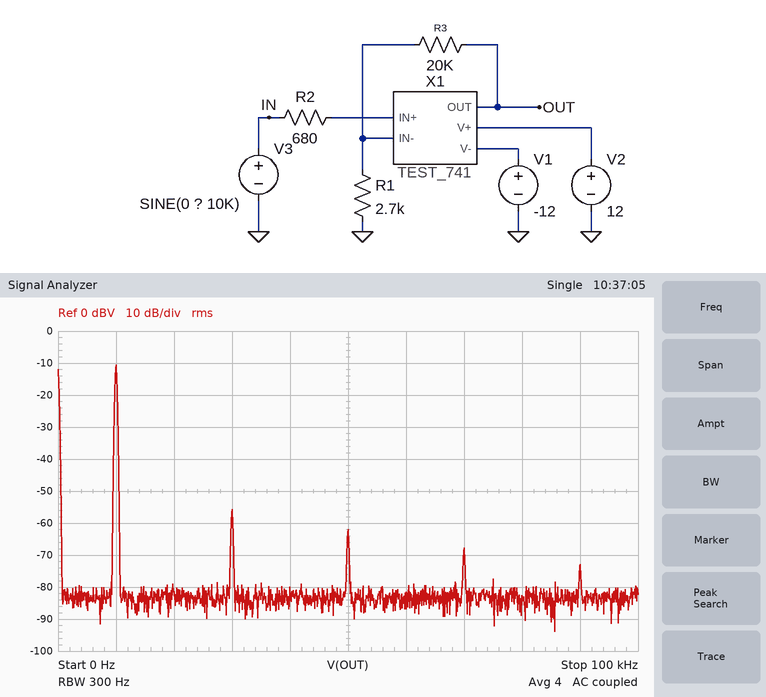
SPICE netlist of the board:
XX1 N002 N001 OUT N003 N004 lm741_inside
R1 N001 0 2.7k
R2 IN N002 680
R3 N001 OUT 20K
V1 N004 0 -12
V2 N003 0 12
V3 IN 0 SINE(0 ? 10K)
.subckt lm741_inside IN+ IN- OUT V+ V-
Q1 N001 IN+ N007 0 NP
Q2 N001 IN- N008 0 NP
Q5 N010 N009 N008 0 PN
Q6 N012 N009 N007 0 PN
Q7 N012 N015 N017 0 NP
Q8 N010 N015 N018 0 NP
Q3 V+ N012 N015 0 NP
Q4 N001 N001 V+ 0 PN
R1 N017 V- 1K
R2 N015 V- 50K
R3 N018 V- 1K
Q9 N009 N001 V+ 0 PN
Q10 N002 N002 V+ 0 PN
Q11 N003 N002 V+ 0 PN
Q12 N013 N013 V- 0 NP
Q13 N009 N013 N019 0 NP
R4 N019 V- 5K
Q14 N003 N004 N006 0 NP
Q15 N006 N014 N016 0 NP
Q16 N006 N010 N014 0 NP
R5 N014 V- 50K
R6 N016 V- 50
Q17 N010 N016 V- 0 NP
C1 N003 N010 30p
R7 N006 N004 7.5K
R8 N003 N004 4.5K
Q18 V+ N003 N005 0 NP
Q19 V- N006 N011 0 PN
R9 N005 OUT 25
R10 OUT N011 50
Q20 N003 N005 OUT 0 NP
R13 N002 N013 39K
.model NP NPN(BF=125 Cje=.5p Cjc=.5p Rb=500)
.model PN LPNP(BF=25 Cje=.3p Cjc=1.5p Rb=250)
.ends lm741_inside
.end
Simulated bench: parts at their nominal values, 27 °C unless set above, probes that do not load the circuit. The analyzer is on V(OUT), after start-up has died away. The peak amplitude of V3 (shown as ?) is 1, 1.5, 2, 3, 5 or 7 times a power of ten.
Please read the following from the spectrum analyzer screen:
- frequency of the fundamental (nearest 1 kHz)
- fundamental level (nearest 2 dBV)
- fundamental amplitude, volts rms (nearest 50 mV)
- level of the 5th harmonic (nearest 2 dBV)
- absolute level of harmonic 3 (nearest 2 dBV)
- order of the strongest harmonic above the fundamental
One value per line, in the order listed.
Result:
10 kHz
-10 dBV
300 mV
-62 dBV
-56 dBV
3
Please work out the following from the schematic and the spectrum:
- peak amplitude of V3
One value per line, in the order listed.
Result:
50 mV
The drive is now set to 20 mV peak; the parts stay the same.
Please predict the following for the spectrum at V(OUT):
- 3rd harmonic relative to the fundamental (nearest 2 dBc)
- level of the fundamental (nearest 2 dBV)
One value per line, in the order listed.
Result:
-48 dBc
-18 dBV
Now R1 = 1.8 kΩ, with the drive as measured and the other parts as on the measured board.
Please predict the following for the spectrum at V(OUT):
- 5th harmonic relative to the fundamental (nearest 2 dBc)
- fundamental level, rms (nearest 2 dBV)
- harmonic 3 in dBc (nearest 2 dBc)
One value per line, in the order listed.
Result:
-48 dBc
-8 dBV
-42 dBc
